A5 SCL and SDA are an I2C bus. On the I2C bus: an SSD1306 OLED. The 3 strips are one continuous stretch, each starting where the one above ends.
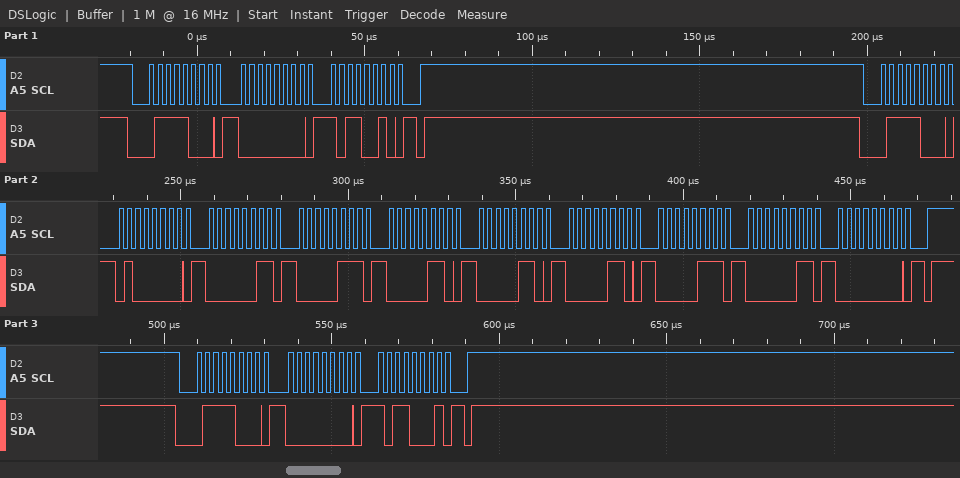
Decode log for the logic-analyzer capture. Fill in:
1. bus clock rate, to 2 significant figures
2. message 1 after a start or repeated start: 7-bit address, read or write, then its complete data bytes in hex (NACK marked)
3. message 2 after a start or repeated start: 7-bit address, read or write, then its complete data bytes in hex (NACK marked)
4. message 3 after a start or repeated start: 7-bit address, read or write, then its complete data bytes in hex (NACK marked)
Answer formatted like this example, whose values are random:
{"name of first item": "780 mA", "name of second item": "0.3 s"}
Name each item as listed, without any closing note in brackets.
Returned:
{"bus clock rate, to 2 significant figures": "400 kHz", "message 1 after a start or repeated start: 7-bit address, read or write, then its complete data bytes in hex": "0x3C write: 00 B2", "message 2 after a start or repeated start: 7-bit address, read or write, then its complete data bytes in hex": "0x3C write: 40 03 07 06 06 06 07 03 00", "message 3 after a start or repeated start: 7-bit address, read or write, then its complete data bytes in hex": "0x3C write: 00 B1"}
